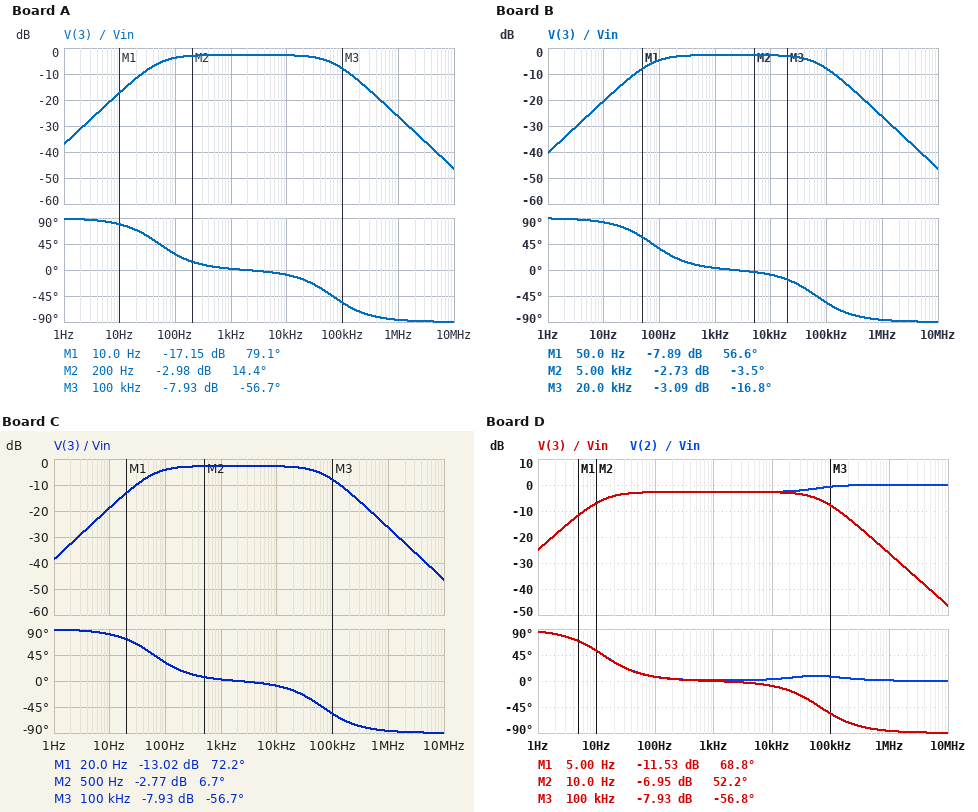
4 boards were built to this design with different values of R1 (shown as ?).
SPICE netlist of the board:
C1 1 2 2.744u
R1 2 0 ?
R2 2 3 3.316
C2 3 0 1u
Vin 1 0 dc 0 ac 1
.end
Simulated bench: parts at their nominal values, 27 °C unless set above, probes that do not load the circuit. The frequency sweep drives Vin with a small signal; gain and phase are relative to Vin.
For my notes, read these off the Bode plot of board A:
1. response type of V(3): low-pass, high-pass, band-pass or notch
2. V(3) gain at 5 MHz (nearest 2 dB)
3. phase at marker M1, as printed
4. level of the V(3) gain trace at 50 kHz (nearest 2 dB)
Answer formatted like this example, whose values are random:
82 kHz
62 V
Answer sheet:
band-pass
-40 dB
79.1 deg
-4 dB
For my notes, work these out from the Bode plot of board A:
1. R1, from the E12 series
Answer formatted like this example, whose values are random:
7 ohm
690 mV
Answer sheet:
820 Ω
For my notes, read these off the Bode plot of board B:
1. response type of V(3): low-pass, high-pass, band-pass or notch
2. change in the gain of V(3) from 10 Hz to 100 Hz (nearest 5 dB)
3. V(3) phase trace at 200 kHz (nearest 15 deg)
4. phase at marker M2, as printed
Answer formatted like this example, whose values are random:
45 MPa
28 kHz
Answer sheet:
band-pass
15 dB
-75 deg
-3.5 deg
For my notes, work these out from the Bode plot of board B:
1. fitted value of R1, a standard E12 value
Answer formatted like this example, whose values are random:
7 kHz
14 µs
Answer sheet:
560 Ω
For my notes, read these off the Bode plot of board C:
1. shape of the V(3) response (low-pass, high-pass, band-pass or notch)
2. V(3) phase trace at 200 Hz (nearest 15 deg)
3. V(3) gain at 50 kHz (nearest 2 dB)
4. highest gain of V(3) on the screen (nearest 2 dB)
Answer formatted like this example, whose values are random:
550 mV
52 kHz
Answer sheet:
band-pass
15 deg
-4 dB
-2 dB
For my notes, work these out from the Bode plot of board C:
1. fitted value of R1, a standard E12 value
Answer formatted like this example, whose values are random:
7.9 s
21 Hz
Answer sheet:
680 Ω
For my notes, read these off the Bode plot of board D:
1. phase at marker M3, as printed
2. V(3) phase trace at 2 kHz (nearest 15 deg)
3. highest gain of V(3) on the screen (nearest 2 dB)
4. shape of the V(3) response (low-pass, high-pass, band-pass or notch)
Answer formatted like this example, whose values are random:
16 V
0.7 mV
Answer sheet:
-56.8 deg
0 deg
-2 dB
band-pass
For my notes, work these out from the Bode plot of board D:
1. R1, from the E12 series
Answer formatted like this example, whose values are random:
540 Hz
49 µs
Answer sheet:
3.3 kΩ
